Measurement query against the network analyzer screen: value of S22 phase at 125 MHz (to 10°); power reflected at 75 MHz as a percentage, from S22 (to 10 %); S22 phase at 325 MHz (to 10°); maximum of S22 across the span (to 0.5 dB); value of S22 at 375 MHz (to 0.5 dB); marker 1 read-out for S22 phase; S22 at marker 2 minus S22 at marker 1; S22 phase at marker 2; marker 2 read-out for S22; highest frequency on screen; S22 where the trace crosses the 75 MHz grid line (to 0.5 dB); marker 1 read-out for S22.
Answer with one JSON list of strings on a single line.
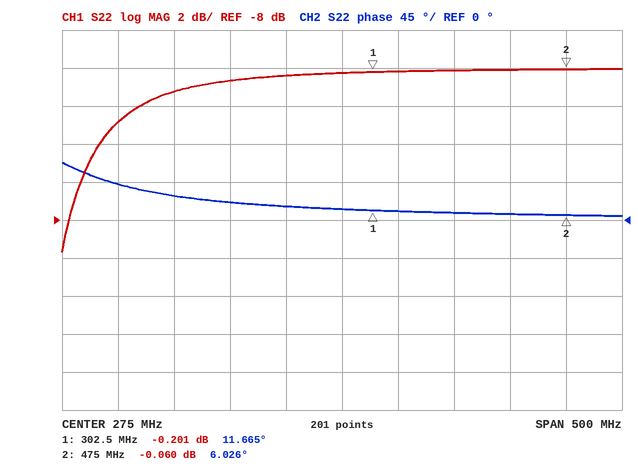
["30°", "50 %", "10°", "0.0 dB", "0.0 dB", "11.665°", "0.141 dB", "6.026°", "-0.060 dB", "525 MHz", "-3.0 dB", "-0.201 dB"]
